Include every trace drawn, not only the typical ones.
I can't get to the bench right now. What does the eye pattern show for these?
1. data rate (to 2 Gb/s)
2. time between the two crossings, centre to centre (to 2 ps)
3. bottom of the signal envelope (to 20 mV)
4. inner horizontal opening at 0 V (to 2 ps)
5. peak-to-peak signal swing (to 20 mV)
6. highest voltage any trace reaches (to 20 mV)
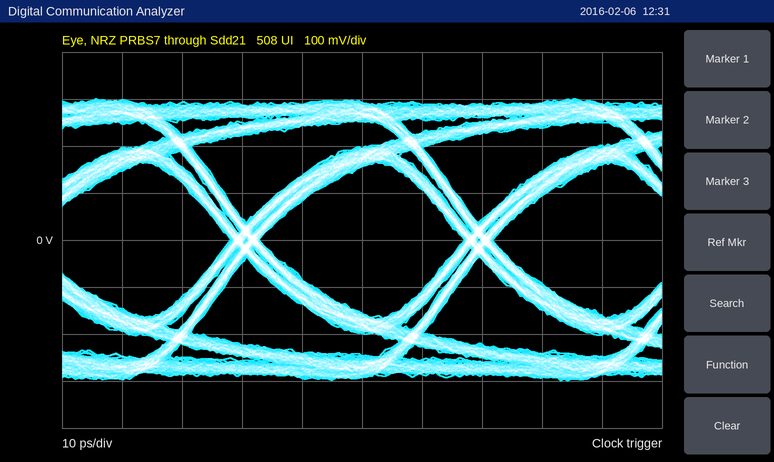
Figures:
26 Gb/s
38 ps
-300 mV
34 ps
600 mV
300 mV
